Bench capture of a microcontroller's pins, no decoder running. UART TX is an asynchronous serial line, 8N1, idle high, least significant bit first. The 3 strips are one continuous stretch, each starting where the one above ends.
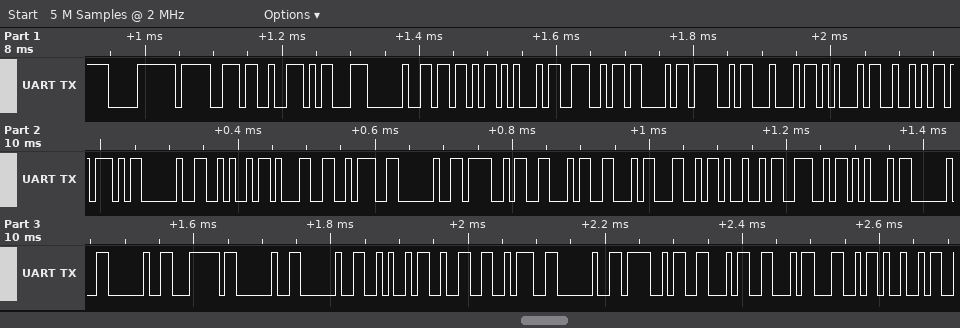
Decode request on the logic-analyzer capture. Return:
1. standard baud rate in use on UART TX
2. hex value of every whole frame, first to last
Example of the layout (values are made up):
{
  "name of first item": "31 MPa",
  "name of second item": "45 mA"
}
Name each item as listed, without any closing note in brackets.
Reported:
{
  "standard baud rate in use on UART TX": "115200 baud",
  "hex value of every whole frame, first to last": "F0 9F 93 8D 20 5B 45 4E 43 4F 44 45 52 5D 20 4A 31 3A 20 4F 46 46 4C 49 4E 45 20 20 7C 20 20 4A 32 3A 20 4F 46 46 4C 49"
}
